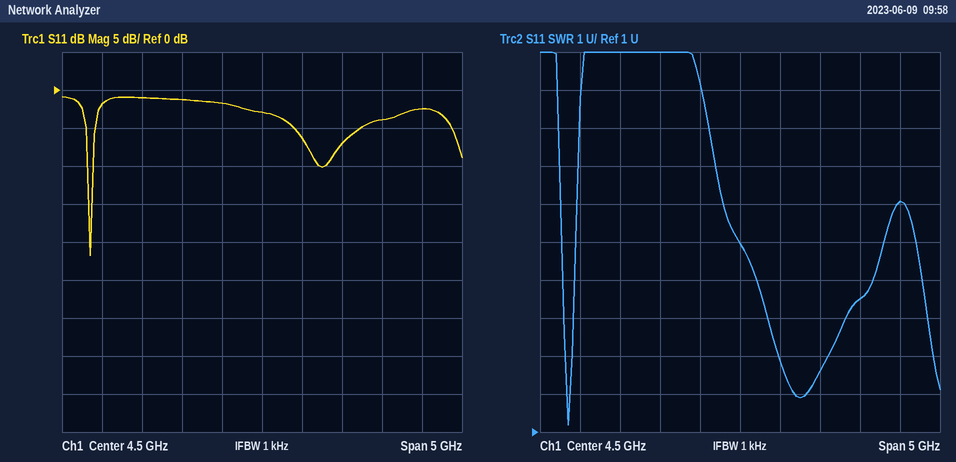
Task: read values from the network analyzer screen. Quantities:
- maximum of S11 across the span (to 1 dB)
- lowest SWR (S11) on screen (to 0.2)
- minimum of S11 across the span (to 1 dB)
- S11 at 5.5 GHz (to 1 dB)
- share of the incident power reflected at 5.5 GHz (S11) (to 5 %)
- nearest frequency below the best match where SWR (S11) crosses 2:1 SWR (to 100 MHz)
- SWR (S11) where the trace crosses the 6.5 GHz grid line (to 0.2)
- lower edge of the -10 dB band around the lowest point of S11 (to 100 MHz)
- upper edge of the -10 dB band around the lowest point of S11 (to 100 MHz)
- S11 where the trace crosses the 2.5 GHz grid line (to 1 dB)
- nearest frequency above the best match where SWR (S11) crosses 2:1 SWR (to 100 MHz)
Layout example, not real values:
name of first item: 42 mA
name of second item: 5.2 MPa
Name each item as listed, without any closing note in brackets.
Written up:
maximum of S11 across the span: -1 dB
lowest SWR (S11) on screen: 1.2
minimum of S11 across the span: -22 dB
S11 at 5.5 GHz: -7 dB
share of the incident power reflected at 5.5 GHz (S11): 20 %
nearest frequency below the best match where SWR (S11) crosses 2:1 SWR: 2.3 GHz
SWR (S11) where the trace crosses the 6.5 GHz grid line: 7.0
lower edge of the -10 dB band around the lowest point of S11: 2.3 GHz
upper edge of the -10 dB band around the lowest point of S11: 2.4 GHz
S11 where the trace crosses the 2.5 GHz grid line: -2 dB
nearest frequency above the best match where SWR (S11) crosses 2:1 SWR: 2.4 GHz
